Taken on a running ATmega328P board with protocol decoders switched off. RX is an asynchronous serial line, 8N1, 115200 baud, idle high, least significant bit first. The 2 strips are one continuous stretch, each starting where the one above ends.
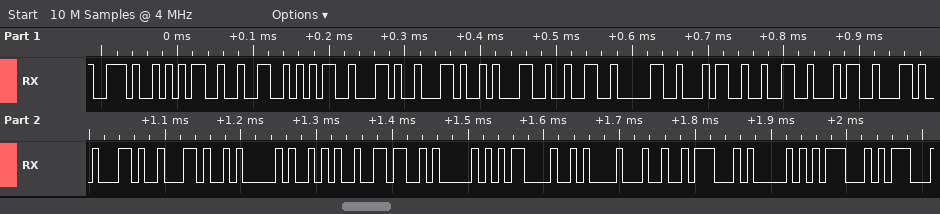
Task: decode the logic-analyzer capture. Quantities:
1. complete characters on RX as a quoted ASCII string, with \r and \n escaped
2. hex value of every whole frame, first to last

".525,,120424,,,A*6A\r\n$GPG"
2E 35 32 35 2C 2C 31 32 30 34 32 34 2C 2C 2C 41 2A 36 41 0D 0A 24 47 50 47
